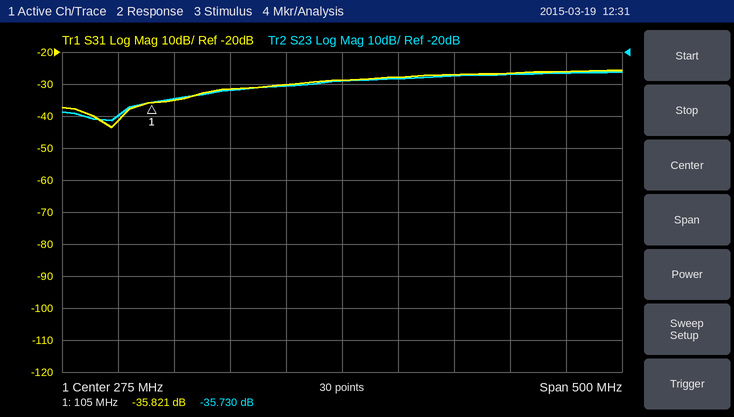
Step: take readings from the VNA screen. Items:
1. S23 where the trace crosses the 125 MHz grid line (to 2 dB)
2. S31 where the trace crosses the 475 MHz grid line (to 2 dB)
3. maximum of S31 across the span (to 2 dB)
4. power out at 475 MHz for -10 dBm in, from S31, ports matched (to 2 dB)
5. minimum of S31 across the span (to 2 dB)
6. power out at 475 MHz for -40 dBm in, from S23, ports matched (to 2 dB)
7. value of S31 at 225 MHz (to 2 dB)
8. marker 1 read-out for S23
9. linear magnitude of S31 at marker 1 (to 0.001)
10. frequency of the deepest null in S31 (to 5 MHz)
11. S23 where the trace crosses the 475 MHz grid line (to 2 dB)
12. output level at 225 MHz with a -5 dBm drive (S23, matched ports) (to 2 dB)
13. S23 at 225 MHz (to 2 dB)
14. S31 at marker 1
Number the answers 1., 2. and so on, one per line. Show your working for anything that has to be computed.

1. -34 dB
2. -26 dB
3. -26 dB
4. -10 dBm + (-26 dB) = -36 dBm
5. -44 dB
6. -40 dBm + (-26 dB) = -66 dBm
7. -30 dB
8. -35.730 dB
9. 10^(-35.821/20) ≈ 0.016
10. 70 MHz
11. -26 dB
12. -5 dBm + (-30 dB) = -36 dBm
13. -30 dB
14. -35.821 dB
